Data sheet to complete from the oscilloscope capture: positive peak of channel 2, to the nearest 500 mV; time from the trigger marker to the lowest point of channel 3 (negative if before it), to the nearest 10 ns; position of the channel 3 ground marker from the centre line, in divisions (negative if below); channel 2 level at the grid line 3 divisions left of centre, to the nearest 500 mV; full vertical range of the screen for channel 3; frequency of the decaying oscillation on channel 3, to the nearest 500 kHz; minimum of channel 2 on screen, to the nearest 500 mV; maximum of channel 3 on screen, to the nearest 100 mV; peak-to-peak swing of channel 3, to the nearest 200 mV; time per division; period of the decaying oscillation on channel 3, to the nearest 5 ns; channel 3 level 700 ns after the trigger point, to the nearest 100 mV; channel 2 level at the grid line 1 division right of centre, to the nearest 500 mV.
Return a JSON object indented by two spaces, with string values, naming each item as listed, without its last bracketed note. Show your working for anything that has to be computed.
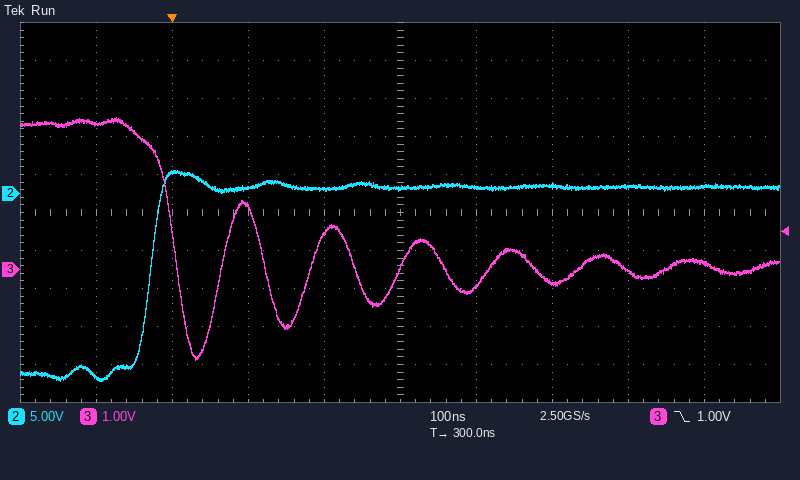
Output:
{
  "positive peak of channel 2, to the nearest 500 mV": "3.0 V",
  "time from the trigger marker to the lowest point of channel 3 (negative if before it), to the nearest 10 ns": "+30 ns",
  "position of the channel 3 ground marker from the centre line, in divisions": "-1.5 div",
  "channel 2 level at the grid line 3 divisions left of centre, to the nearest 500 mV": "2.5 V",
  "full vertical range of the screen for channel 3": "10 V",
  "frequency of the decaying oscillation on channel 3, to the nearest 500 kHz": "1 / 120 ns ≈ 8.33 MHz, so 8.5 MHz to the nearest 500 kHz",
  "minimum of channel 2 on screen, to the nearest 500 mV": "-24.5 V",
  "maximum of channel 3 on screen, to the nearest 100 mV": "4.0 V",
  "peak-to-peak swing of channel 3, to the nearest 200 mV": "6.4 V",
  "time per division": "100 ns",
  "period of the decaying oscillation on channel 3, to the nearest 5 ns": "120 ns",
  "channel 3 level 700 ns after the trigger point, to the nearest 100 mV": "200 mV",
  "channel 2 level at the grid line 1 division right of centre, to the nearest 500 mV": "1.0 V"
}
